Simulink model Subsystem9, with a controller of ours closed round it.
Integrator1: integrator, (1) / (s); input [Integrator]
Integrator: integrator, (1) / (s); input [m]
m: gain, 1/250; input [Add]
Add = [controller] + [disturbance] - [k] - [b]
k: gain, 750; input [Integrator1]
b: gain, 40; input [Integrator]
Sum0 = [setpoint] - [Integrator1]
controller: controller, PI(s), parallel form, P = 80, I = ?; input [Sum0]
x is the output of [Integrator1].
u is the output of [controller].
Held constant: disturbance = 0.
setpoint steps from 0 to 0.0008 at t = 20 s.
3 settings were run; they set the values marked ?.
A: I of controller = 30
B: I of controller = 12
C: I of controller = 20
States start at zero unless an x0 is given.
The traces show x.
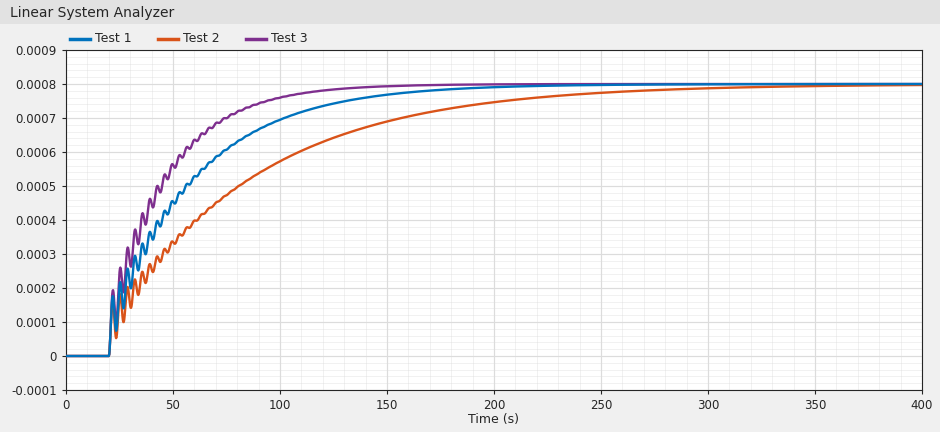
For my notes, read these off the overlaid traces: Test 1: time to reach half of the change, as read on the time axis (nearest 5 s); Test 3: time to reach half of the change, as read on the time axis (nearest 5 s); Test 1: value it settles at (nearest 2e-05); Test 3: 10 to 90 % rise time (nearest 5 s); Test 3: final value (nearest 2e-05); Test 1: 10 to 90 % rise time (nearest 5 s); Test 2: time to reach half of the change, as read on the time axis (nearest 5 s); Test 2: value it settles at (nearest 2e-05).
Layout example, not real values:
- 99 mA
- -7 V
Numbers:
- 45 s
- 35 s
- 0.00080
- 60 s
- 0.00080
- 90 s
- 60 s
- 0.00080
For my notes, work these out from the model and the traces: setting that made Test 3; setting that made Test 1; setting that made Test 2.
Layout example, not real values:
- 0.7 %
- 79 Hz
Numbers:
- A
- C
- B
